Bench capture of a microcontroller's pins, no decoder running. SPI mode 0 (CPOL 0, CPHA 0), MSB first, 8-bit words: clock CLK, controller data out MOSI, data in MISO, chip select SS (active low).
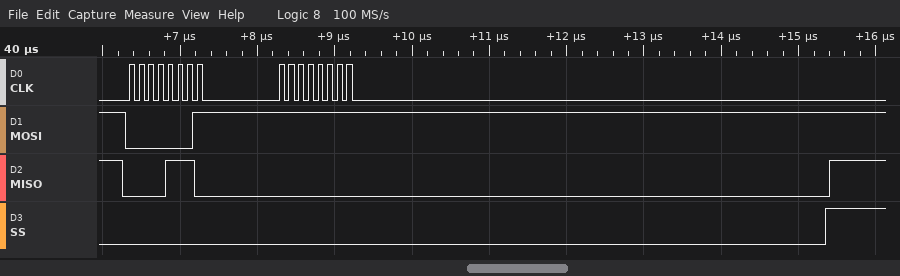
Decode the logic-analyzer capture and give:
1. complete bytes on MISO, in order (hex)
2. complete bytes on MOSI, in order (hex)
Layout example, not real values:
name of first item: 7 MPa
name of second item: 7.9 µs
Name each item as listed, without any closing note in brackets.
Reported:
complete bytes on MISO, in order: 0E 00
complete bytes on MOSI, in order: 01 FF
